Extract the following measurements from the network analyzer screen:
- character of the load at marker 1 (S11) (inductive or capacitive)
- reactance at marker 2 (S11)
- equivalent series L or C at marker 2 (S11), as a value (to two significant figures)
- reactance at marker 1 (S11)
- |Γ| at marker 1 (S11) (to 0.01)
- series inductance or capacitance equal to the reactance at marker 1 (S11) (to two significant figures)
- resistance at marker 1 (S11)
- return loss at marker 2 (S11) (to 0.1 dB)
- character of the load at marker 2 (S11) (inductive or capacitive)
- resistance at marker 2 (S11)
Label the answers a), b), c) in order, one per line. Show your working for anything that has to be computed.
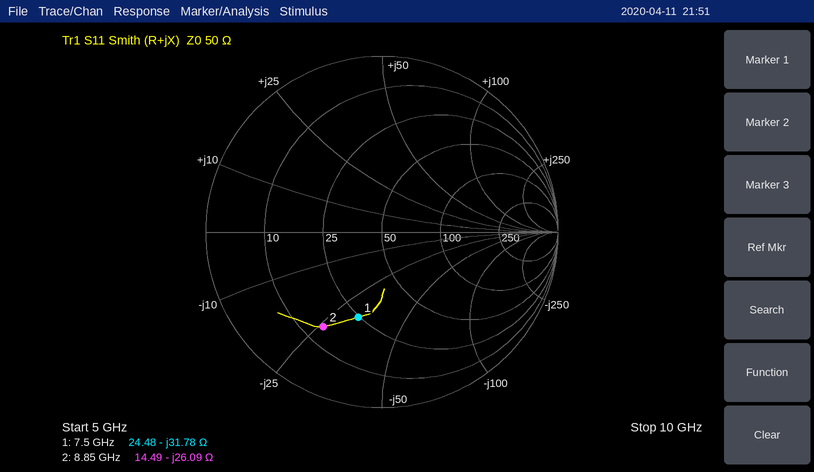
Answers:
a) capacitive
b) -26.09 Ω
c) C = 1/(2π × 8.85 GHz × 26.09 Ω) ≈ 689 fF, so 690 fF to two significant figures
d) -31.78 Ω
e) 0.50
f) C = 1/(2π × 7.5 GHz × 31.78 Ω) ≈ 668 fF, so 670 fF to two significant figures
g) 24.48 Ω
h) 4.0 dB
i) capacitive
j) 14.49 Ω
